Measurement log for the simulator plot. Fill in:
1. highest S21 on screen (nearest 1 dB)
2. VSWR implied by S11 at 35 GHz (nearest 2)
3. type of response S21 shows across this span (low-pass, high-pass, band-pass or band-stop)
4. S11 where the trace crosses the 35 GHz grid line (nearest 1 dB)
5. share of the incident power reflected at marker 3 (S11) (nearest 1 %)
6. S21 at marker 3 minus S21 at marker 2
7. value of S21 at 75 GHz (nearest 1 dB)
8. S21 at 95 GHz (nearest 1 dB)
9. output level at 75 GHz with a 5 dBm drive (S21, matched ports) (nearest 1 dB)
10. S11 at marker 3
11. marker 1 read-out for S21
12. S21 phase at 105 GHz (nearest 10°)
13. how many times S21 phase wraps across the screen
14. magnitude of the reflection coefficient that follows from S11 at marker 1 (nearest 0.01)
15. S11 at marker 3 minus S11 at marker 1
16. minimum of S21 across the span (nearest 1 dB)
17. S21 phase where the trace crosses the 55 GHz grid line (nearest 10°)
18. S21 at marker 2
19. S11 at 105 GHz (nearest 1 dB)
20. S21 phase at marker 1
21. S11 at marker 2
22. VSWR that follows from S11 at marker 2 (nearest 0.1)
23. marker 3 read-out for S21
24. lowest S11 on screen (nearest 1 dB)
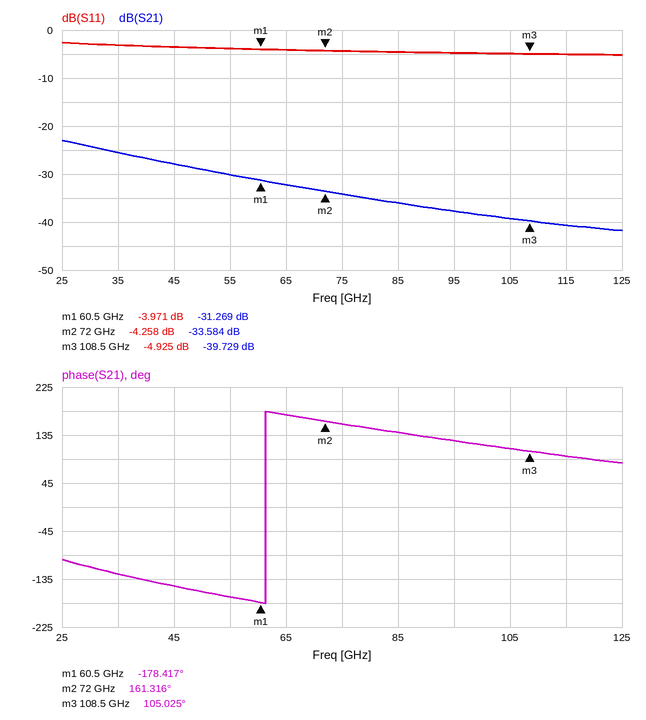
-23 dB
6
low-pass
-3 dB
32 %
-6.145 dB
-34 dB
-38 dB
-29 dBm
-4.925 dB
-31.269 dB
110°
1
0.63
-0.954 dB
-42 dB
-170°
-33.584 dB
-5 dB
-178.417°
-4.258 dB
4.2
-39.729 dB
-5 dB
